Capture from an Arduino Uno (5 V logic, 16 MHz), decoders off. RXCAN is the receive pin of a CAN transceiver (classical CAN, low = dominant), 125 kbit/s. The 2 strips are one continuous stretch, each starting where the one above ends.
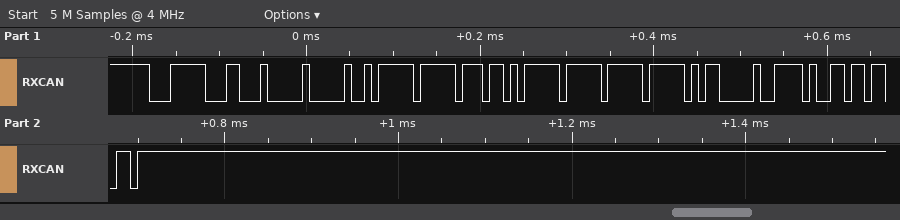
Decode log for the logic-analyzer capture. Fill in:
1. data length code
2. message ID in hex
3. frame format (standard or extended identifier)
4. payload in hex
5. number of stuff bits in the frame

8
0x1F3
standard
00 5F FF 6B FF FF EC 07
10
